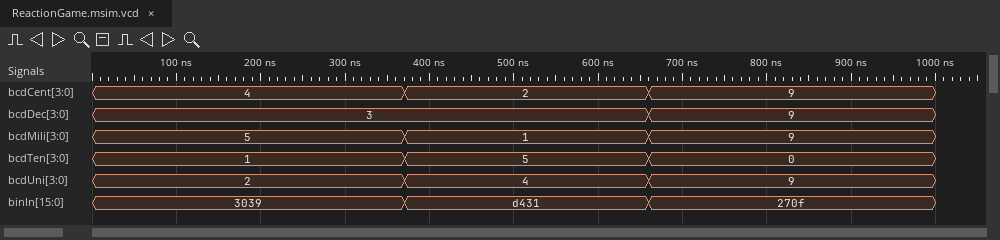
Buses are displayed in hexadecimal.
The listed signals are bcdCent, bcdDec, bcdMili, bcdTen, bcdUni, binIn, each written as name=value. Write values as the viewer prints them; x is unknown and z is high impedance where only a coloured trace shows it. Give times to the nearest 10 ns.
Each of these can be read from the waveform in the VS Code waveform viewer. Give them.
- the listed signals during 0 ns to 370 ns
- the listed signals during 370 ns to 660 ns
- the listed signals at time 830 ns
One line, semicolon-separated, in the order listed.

bcdCent=4, bcdDec=3, bcdMili=5, bcdTen=1, bcdUni=2, binIn=3039; bcdCent=2, bcdDec=3, bcdMili=1, bcdTen=5, bcdUni=4, binIn=d431; bcdCent=9, bcdDec=9, bcdMili=9, bcdTen=0, bcdUni=9, binIn=270f
